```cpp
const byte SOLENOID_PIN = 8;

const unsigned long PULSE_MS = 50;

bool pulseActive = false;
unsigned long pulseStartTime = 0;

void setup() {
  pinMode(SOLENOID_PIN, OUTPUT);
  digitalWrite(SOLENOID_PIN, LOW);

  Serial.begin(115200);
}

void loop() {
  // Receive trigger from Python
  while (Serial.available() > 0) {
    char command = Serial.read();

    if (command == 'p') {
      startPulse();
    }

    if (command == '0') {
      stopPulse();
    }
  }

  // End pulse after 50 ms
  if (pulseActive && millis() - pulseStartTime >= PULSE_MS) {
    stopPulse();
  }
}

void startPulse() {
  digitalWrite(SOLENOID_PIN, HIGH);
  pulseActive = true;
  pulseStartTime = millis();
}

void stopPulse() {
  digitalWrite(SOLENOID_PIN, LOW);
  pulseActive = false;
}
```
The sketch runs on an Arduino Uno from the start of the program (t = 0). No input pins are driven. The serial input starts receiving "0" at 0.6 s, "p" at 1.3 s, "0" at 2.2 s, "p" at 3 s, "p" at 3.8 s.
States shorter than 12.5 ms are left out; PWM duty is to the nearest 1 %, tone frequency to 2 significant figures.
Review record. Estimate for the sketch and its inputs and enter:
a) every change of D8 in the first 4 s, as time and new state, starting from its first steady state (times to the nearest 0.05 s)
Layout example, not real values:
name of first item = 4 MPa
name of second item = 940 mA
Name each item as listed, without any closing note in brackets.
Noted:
every change of D8 in the first 4 s, as time and new state, starting from its first steady state = 0 s low; 1.3 s high; 1.35 s low; 3 s high; 3.05 s low; 3.8 s high; 3.85 s low
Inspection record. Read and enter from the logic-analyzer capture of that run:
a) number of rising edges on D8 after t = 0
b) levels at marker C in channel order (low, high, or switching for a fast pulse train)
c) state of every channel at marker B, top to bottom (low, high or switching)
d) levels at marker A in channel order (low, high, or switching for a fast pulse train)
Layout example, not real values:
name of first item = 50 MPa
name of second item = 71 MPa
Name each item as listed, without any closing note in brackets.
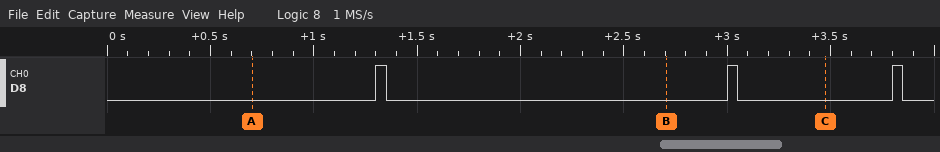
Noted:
number of rising edges on D8 after t = 0 = 3
levels at marker C in channel order = D8 low
state of every channel at marker B, top to bottom = D8 low
levels at marker A in channel order = D8 low
